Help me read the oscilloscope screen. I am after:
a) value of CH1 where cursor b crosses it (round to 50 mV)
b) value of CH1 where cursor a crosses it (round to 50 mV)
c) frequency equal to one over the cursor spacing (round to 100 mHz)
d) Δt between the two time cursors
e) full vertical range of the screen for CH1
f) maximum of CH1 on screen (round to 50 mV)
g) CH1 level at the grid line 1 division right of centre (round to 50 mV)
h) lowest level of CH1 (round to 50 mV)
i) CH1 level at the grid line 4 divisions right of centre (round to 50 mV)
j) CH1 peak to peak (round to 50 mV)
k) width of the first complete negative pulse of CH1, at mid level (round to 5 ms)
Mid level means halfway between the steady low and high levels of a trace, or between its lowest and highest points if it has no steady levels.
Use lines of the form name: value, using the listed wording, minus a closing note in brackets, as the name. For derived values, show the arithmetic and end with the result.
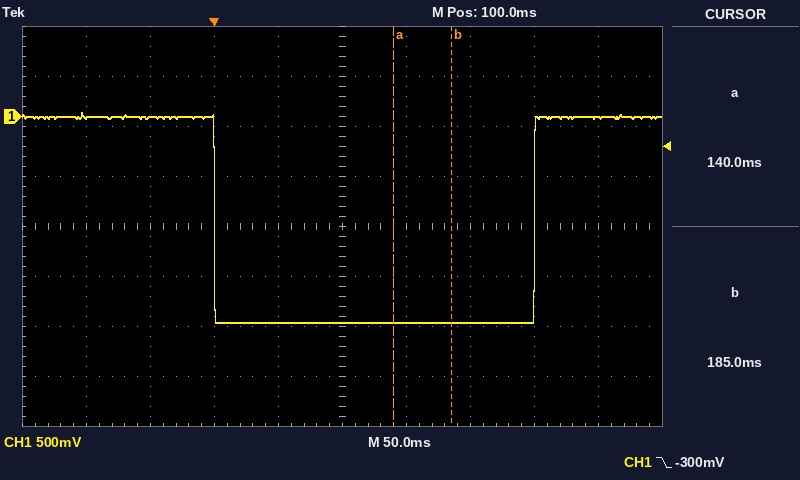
value of CH1 where cursor b crosses it: -2.05 V
value of CH1 where cursor a crosses it: -2.05 V
frequency equal to one over the cursor spacing: 1 / 45 ms ≈ 22.2 Hz
Δt between the two time cursors: 185 ms − (140 ms) = 45 ms
full vertical range of the screen for CH1: 4 V
maximum of CH1 on screen: 50 mV
CH1 level at the grid line 1 division right of centre: -2.05 V
lowest level of CH1: -2.05 V
CH1 level at the grid line 4 divisions right of centre: 0 mV
CH1 peak to peak: 50 mV − (-2.05 V) = 2.10 V
width of the first complete negative pulse of CH1, at mid level: 250 ms
